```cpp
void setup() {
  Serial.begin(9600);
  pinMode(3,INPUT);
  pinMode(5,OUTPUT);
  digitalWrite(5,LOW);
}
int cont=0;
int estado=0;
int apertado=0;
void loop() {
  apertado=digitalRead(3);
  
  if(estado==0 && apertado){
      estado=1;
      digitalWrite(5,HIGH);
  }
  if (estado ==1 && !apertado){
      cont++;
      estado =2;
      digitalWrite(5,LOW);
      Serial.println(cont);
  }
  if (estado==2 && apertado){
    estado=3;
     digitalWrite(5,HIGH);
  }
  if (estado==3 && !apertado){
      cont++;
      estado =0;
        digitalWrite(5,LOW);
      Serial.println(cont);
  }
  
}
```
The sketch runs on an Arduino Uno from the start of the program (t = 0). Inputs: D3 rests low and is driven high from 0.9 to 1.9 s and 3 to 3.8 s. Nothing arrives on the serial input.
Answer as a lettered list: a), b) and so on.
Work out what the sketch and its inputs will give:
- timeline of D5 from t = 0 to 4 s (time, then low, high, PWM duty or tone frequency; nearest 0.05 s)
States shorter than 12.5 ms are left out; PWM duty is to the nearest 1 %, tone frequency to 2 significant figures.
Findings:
a) 0 s low; 0.9 s high; 1.9 s low; 3 s high; 3.8 s low
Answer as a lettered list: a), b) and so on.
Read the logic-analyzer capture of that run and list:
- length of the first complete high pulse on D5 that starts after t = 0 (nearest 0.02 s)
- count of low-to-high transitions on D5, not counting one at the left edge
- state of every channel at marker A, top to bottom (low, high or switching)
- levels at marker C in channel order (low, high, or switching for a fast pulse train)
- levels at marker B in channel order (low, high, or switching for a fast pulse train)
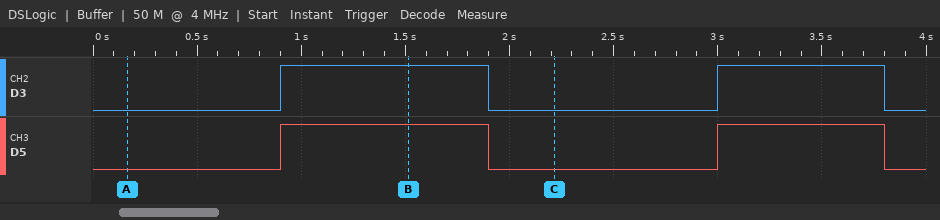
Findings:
a) 1.00 s
b) 2
c) D3 low, D5 low
d) D3 low, D5 low
e) D3 high, D5 high
